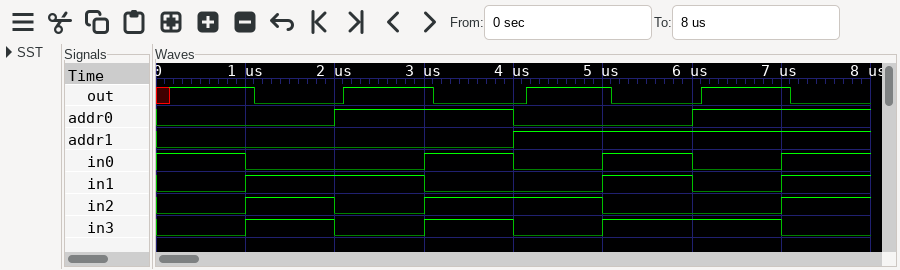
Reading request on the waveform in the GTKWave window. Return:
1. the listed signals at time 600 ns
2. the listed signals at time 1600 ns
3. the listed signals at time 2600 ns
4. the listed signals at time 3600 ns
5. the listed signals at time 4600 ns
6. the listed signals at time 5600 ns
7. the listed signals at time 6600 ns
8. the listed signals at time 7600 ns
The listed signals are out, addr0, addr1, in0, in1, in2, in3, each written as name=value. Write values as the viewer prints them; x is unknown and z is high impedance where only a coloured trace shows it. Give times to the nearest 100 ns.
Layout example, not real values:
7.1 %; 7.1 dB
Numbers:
out=1, addr0=0, addr1=0, in0=1, in1=0, in2=0, in3=0; out=0, addr0=0, addr1=0, in0=0, in1=1, in2=1, in3=1; out=1, addr0=1, addr1=0, in0=0, in1=1, in2=0, in3=0; out=0, addr0=1, addr1=0, in0=1, in1=0, in2=1, in3=1; out=1, addr0=0, addr1=1, in0=0, in1=0, in2=1, in3=0; out=0, addr0=0, addr1=1, in0=1, in1=1, in2=0, in3=1; out=1, addr0=1, addr1=1, in0=0, in1=0, in2=0, in3=1; out=0, addr0=1, addr1=1, in0=1, in1=1, in2=1, in3=0
